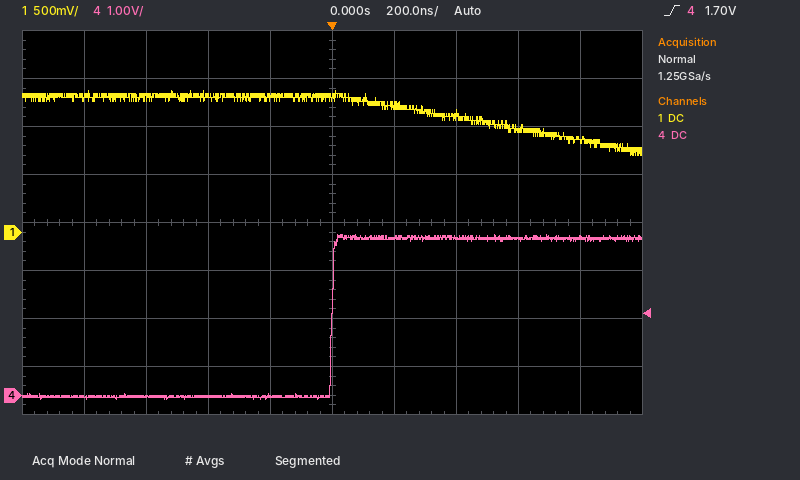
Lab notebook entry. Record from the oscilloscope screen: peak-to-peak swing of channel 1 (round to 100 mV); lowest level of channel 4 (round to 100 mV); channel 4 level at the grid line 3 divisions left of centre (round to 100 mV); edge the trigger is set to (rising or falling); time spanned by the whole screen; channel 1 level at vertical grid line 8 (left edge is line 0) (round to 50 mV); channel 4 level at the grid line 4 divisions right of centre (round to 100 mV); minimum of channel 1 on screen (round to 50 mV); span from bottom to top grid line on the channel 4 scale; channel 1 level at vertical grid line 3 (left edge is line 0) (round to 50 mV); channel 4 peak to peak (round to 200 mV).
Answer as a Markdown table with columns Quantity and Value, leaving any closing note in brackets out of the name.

| Quantity | Value |
|---|---|
| peak-to-peak swing of channel 1 | 700 mV |
| lowest level of channel 4 | -100 mV |
| channel 4 level at the grid line 3 divisions left of centre | 0.0 V |
| edge the trigger is set to | rising |
| time spanned by the whole screen | 2 µs |
| channel 1 level at vertical grid line 8 (left edge is line 0) | 1.10 V |
| channel 4 level at the grid line 4 divisions right of centre | 3.3 V |
| minimum of channel 1 on screen | 800 mV |
| span from bottom to top grid line on the channel 4 scale | 8 V |
| channel 1 level at vertical grid line 3 (left edge is line 0) | 1.40 V |
| channel 4 peak to peak | 3.4 V |
